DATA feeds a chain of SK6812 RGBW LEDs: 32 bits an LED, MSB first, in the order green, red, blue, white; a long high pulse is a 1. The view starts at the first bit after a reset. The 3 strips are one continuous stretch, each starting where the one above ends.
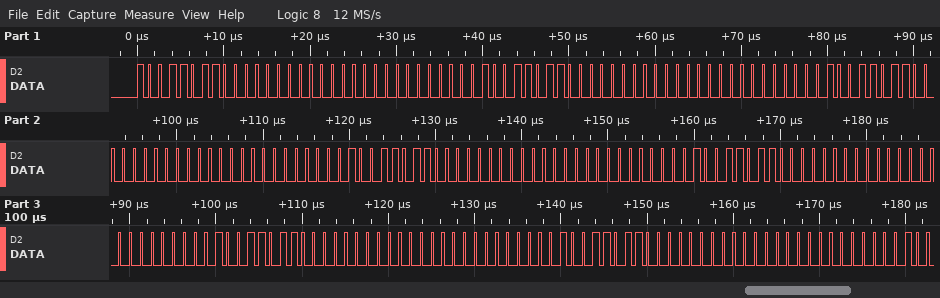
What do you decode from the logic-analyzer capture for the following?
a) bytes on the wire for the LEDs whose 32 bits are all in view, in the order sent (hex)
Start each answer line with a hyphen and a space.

- 9B 00 00 00 9B 00 00 00 9B 00 00 00 9B 00 00 00 9B 00 00 00 9B 00 00 00 9B 00 00 00
